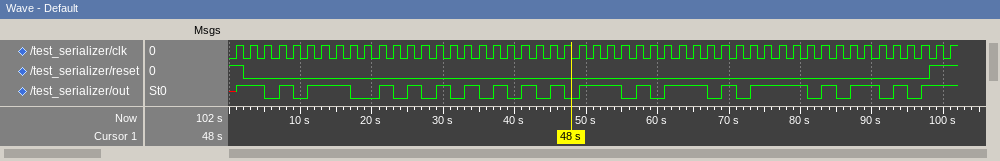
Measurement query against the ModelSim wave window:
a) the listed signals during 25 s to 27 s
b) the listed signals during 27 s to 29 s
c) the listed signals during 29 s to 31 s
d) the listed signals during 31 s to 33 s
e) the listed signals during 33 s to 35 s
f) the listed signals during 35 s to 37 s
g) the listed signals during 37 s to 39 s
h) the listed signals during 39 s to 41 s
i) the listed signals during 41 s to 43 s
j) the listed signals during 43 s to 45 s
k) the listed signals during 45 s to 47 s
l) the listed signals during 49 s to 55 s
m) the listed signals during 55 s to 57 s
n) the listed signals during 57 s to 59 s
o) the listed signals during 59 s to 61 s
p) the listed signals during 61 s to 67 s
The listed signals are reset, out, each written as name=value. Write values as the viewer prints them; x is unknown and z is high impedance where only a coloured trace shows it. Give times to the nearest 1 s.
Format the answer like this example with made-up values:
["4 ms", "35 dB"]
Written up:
["reset=0, out=1", "reset=0, out=0", "reset=0, out=1", "reset=0, out=0", "reset=0, out=1", "reset=0, out=0", "reset=0, out=1", "reset=0, out=0", "reset=0, out=1", "reset=0, out=0", "reset=0, out=1", "reset=0, out=1", "reset=0, out=0", "reset=0, out=1", "reset=0, out=0", "reset=0, out=1"]
